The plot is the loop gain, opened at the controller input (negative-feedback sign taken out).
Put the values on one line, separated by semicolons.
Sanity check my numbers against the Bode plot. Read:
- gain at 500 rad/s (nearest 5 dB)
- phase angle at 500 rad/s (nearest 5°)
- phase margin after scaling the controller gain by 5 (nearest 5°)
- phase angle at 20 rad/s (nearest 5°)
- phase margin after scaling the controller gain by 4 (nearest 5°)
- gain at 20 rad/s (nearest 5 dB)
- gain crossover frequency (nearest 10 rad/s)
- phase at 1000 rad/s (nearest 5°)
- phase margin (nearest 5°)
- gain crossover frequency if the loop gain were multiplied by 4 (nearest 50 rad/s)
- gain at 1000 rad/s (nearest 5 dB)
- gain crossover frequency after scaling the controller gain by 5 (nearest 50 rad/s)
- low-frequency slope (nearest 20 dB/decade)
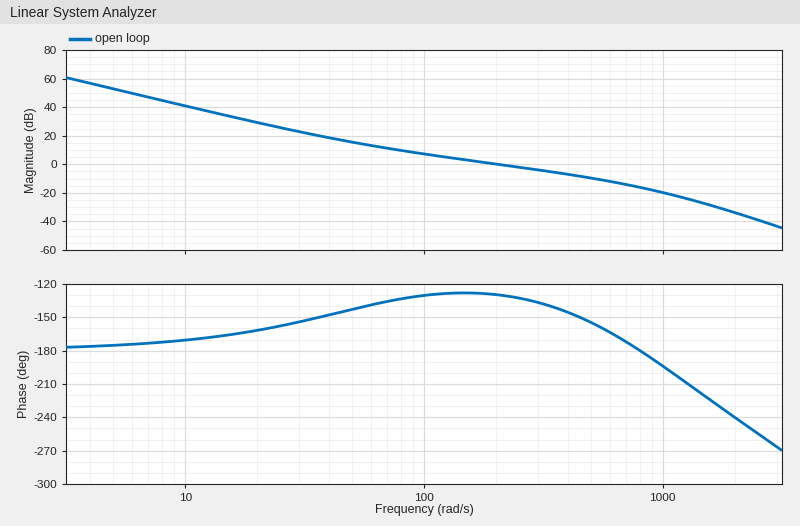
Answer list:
-10 dB; -155°; 10°; -160°; 15°; 30 dB; 200 rad/s; -195°; 50°; 600 rad/s; -20 dB; 700 rad/s; -40 dB/decade
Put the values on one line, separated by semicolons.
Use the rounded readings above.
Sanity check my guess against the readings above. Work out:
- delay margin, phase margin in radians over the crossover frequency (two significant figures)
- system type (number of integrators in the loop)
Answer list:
0.0044 s; 2
